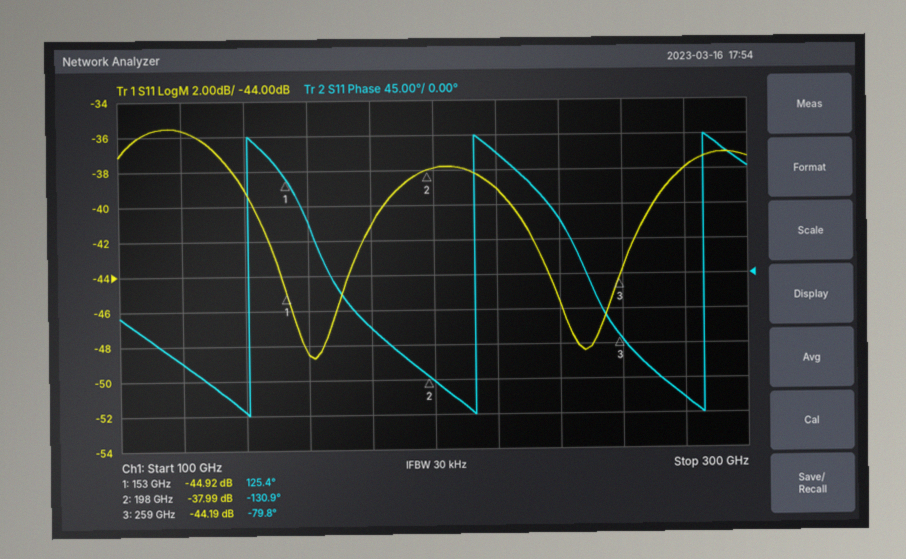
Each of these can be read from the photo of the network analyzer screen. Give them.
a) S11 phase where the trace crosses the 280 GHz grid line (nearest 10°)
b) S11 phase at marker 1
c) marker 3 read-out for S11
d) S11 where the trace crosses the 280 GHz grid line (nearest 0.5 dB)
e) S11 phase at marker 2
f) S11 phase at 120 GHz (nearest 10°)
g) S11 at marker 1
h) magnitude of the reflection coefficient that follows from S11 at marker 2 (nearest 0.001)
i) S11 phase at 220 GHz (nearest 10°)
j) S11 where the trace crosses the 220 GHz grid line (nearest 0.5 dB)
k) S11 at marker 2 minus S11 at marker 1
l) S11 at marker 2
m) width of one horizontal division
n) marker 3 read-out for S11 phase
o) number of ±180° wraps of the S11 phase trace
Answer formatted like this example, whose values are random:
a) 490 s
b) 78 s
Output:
a) -160°
b) 125.4°
c) -44.19 dB
d) -38.0 dB
e) -130.9°
f) -110°
g) -44.92 dB
h) 0.013
i) 160°
j) -39.0 dB
k) 6.93 dB
l) -37.99 dB
m) 20 GHz
n) -79.8°
o) 3
